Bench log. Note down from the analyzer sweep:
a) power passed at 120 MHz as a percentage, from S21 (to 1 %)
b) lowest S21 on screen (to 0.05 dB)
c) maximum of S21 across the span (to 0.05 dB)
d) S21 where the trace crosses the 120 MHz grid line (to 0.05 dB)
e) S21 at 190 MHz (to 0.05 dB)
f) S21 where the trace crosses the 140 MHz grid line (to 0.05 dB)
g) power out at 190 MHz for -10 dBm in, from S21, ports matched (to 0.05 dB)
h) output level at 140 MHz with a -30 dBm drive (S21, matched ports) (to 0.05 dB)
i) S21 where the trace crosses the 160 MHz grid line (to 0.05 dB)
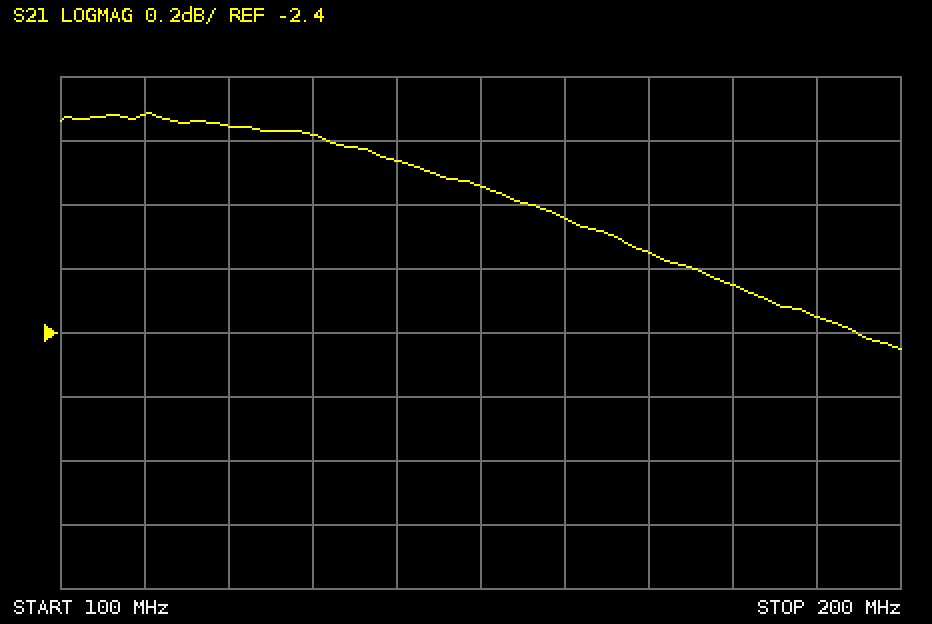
67 %
-2.45 dB
-1.70 dB
-1.75 dB
-2.35 dB
-1.85 dB
-12.35 dBm
-31.85 dBm
-2.05 dB
